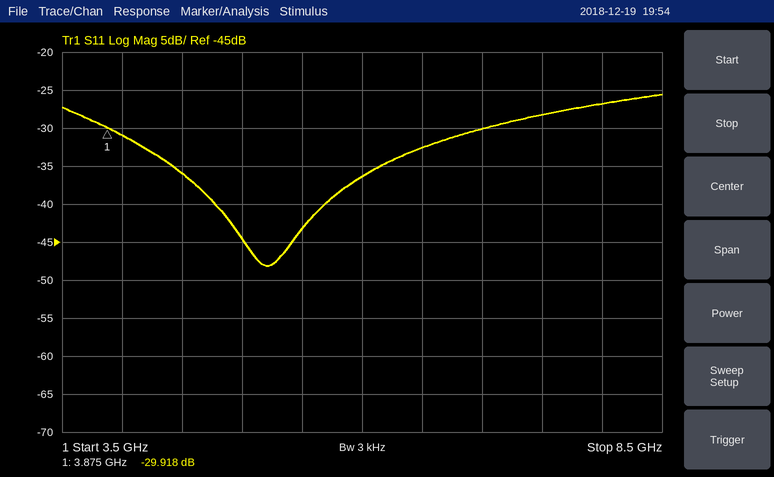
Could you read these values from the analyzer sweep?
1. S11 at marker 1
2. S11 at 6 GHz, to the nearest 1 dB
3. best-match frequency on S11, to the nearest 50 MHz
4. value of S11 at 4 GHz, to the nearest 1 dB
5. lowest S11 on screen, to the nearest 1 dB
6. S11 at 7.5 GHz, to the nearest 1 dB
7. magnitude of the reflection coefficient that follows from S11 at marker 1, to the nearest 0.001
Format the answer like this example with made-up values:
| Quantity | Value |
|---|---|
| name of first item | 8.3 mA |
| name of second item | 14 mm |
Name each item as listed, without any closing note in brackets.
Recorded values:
| Quantity | Value |
|---|---|
| S11 at marker 1 | -29.918 dB |
| S11 at 6 GHz, to the nearest 1 dB | -36 dB |
| best-match frequency on S11, to the nearest 50 MHz | 5.20 GHz |
| value of S11 at 4 GHz, to the nearest 1 dB | -31 dB |
| lowest S11 on screen, to the nearest 1 dB | -48 dB |
| S11 at 7.5 GHz, to the nearest 1 dB | -28 dB |
| magnitude of the reflection coefficient that follows from S11 at marker 1, to the nearest 0.001 | 0.032 |
